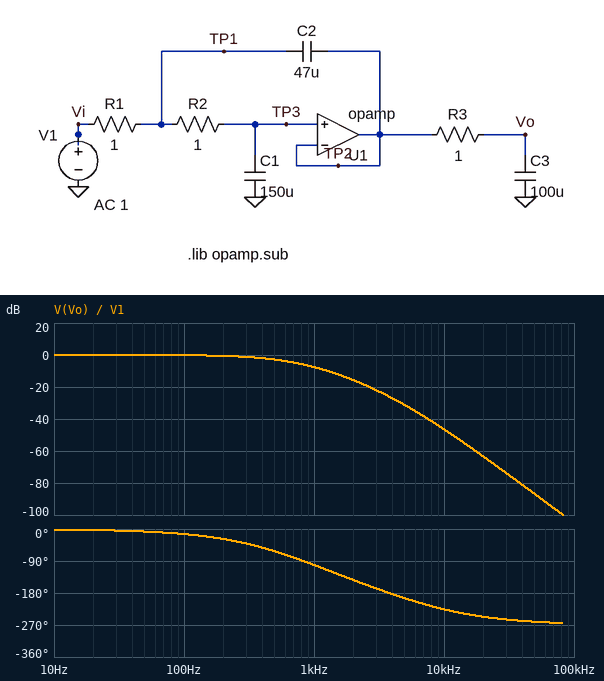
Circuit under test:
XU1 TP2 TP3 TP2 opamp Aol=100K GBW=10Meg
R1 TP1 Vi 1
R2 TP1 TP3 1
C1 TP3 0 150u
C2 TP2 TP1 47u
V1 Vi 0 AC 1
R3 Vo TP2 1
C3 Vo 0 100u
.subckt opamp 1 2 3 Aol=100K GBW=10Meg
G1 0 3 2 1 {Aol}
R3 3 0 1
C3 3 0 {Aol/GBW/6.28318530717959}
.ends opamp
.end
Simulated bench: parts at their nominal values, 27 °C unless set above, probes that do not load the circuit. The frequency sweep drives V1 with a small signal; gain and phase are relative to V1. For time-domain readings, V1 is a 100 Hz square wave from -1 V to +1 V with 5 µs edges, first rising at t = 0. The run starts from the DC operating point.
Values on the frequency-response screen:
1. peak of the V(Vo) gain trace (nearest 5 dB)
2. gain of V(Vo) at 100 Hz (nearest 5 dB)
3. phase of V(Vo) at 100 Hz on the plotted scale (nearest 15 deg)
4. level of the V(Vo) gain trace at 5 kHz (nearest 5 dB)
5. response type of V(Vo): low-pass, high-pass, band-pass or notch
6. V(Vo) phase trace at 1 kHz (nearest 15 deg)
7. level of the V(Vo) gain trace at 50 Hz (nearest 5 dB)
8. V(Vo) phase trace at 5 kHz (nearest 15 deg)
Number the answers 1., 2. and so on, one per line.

1. 0 dB
2. 0 dB
3. -15 deg
4. -30 dB
5. low-pass
6. -105 deg
7. 0 dB
8. -195 deg
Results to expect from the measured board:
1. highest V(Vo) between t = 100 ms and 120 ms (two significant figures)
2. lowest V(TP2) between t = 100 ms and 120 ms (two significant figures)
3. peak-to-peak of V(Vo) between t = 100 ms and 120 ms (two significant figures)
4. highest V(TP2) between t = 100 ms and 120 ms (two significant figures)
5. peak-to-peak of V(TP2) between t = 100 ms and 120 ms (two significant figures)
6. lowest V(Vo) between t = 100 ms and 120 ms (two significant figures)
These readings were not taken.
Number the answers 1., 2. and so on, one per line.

1. 1.0 V
2. -1.0 V
3. 2.0 V
4. 1.0 V
5. 2.0 V
6. -1.0 V
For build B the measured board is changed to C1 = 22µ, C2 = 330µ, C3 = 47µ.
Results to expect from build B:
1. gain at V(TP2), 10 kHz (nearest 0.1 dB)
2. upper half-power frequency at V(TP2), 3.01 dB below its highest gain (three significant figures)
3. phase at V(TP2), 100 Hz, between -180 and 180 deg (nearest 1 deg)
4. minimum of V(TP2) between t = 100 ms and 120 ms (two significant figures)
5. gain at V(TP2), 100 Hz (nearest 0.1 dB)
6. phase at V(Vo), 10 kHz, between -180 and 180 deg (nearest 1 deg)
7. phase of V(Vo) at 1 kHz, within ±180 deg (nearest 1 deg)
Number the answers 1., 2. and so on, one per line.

1. -28.9 dB
2. 2.18 kHz
3. -2 deg
4. -1.9 V
5. 0 dB
6. 114 deg
7. -38 deg
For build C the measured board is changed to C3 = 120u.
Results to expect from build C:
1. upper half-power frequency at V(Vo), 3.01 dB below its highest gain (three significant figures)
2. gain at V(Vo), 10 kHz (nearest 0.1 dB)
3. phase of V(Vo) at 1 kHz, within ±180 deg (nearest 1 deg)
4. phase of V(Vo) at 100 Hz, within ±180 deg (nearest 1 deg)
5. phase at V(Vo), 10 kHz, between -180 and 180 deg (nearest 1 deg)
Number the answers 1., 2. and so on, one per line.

1. 499 Hz
2. -47.9 dB
3. -106 deg
4. -15 deg
5. 133 deg
